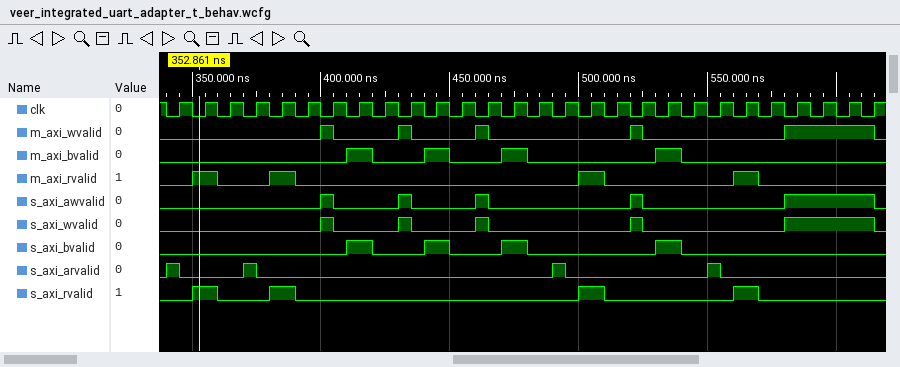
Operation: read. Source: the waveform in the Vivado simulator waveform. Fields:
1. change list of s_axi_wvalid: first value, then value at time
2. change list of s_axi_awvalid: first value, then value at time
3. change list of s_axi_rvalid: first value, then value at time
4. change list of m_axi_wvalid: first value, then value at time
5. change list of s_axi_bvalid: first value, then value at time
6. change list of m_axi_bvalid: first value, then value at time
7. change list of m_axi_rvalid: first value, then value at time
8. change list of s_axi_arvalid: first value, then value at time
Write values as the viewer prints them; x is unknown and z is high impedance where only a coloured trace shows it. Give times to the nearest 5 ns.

0, 1 at 400 ns, 0 at 405 ns, 1 at 430 ns, 0 at 435 ns, 1 at 460 ns, 0 at 465 ns, 1 at 520 ns, 0 at 525 ns, 1 at 580 ns, 0 at 615 ns
0, 1 at 400 ns, 0 at 405 ns, 1 at 430 ns, 0 at 435 ns, 1 at 460 ns, 0 at 465 ns, 1 at 520 ns, 0 at 525 ns, 1 at 580 ns, 0 at 615 ns
0, 1 at 350 ns, 0 at 360 ns, 1 at 380 ns, 0 at 390 ns, 1 at 500 ns, 0 at 510 ns, 1 at 560 ns, 0 at 570 ns
0, 1 at 400 ns, 0 at 405 ns, 1 at 430 ns, 0 at 435 ns, 1 at 460 ns, 0 at 465 ns, 1 at 520 ns, 0 at 525 ns, 1 at 580 ns, 0 at 615 ns
0, 1 at 410 ns, 0 at 420 ns, 1 at 440 ns, 0 at 450 ns, 1 at 470 ns, 0 at 480 ns, 1 at 530 ns, 0 at 540 ns
0, 1 at 410 ns, 0 at 420 ns, 1 at 440 ns, 0 at 450 ns, 1 at 470 ns, 0 at 480 ns, 1 at 530 ns, 0 at 540 ns
0, 1 at 350 ns, 0 at 360 ns, 1 at 380 ns, 0 at 390 ns, 1 at 500 ns, 0 at 510 ns, 1 at 560 ns, 0 at 570 ns
0, 1 at 340 ns, 0 at 345 ns, 1 at 370 ns, 0 at 375 ns, 1 at 490 ns, 0 at 495 ns, 1 at 550 ns, 0 at 555 ns
